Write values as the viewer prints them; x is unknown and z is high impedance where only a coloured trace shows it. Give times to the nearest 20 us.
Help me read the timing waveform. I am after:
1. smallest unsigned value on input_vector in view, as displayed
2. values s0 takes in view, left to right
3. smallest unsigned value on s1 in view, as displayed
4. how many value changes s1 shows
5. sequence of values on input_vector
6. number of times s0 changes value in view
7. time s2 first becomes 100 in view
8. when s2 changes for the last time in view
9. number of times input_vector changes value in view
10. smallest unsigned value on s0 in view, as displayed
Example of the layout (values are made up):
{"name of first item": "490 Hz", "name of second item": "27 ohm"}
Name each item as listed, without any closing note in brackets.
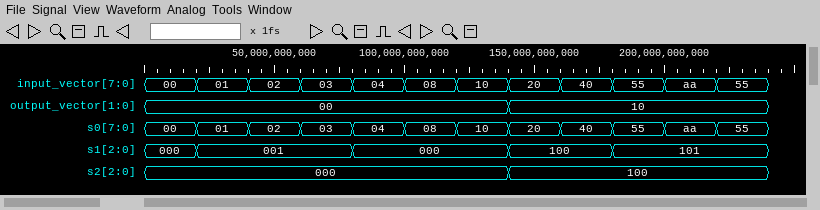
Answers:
{"smallest unsigned value on input_vector in view, as displayed": "00", "values s0 takes in view, left to right": "00, 01, 02, 03, 04, 08, 10, 20, 40, 55, aa, 55", "smallest unsigned value on s1 in view, as displayed": "000", "how many value changes s1 shows": "4", "sequence of values on input_vector": "00, 01, 02, 03, 04, 08, 10, 20, 40, 55, aa, 55", "number of times s0 changes value in view": "11", "time s2 first becomes 100 in view": "140 us", "when s2 changes for the last time in view": "140 us", "number of times input_vector changes value in view": "11", "smallest unsigned value on s0 in view, as displayed": "00"}
